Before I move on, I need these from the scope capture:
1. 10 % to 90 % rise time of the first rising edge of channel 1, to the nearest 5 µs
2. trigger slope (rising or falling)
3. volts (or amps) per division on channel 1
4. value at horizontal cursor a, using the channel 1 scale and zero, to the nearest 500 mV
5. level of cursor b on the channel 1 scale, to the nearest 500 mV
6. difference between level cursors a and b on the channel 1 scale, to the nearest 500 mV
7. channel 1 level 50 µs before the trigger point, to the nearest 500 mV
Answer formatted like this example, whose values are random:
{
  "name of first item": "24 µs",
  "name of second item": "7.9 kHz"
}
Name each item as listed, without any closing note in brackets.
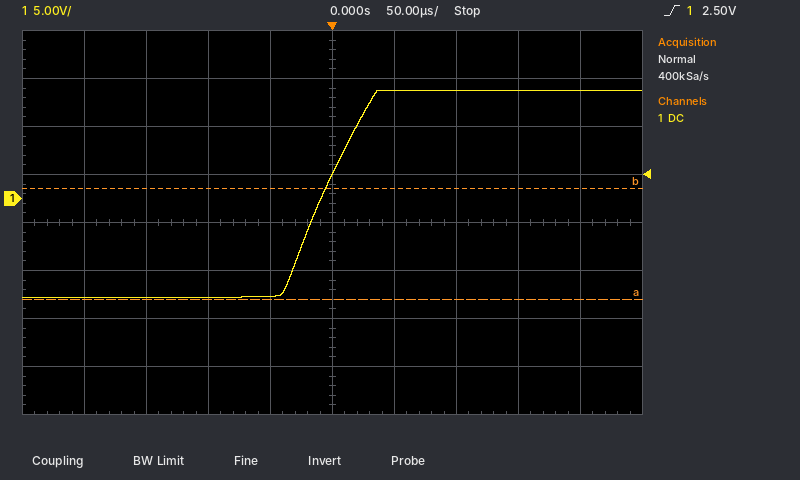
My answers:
{
  "10 % to 90 % rise time of the first rising edge of channel 1, to the nearest 5 µs": "60 µs",
  "trigger slope": "rising",
  "volts (or amps) per division on channel 1": "5 V",
  "value at horizontal cursor a, using the channel 1 scale and zero, to the nearest 500 mV": "-10.5 V",
  "level of cursor b on the channel 1 scale, to the nearest 500 mV": "1.0 V",
  "difference between level cursors a and b on the channel 1 scale, to the nearest 500 mV": "11.5 V",
  "channel 1 level 50 µs before the trigger point, to the nearest 500 mV": "-10.0 V"
}
